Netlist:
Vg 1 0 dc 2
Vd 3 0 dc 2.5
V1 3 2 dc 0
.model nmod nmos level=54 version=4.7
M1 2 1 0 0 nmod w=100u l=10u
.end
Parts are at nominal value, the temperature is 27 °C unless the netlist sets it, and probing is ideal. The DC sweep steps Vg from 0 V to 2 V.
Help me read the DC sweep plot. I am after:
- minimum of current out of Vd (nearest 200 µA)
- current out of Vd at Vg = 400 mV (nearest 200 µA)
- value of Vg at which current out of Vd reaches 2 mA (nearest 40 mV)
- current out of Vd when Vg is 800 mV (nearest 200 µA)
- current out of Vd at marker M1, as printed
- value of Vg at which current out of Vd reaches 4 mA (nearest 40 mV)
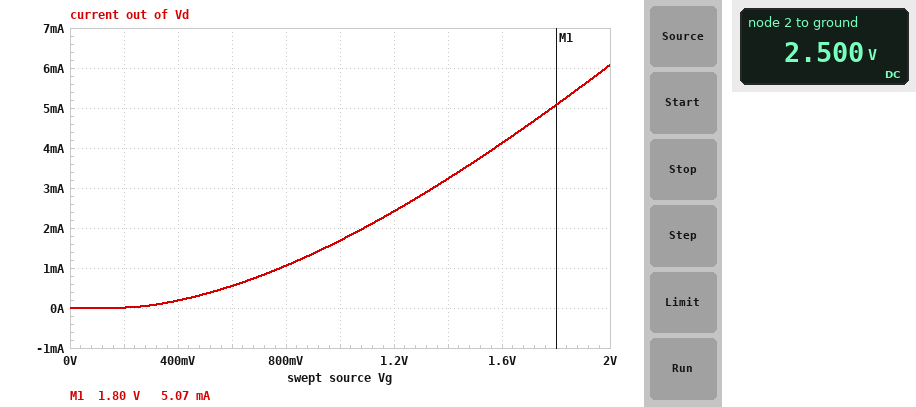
0 A
200 µA
1.08 V
1.0 mA
5.07 mA
1.56 V
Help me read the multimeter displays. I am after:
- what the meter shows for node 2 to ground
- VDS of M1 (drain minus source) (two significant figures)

2.500 V
2.5 V
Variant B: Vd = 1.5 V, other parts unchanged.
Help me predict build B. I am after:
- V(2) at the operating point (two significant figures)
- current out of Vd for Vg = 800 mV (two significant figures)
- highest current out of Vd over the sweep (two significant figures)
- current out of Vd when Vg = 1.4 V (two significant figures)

1.5 V
1.0 mA
5.9 mA
3.2 mA
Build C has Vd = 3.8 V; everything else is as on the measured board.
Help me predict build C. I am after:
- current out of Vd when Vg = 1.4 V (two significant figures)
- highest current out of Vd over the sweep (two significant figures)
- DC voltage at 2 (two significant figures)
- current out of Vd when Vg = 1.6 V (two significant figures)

3.3 mA
6.2 mA
3.8 V
4.2 mA
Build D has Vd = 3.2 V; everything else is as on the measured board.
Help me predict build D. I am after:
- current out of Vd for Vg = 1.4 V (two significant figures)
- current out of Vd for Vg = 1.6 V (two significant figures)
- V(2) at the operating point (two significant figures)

3.3 mA
4.2 mA
3.2 V
